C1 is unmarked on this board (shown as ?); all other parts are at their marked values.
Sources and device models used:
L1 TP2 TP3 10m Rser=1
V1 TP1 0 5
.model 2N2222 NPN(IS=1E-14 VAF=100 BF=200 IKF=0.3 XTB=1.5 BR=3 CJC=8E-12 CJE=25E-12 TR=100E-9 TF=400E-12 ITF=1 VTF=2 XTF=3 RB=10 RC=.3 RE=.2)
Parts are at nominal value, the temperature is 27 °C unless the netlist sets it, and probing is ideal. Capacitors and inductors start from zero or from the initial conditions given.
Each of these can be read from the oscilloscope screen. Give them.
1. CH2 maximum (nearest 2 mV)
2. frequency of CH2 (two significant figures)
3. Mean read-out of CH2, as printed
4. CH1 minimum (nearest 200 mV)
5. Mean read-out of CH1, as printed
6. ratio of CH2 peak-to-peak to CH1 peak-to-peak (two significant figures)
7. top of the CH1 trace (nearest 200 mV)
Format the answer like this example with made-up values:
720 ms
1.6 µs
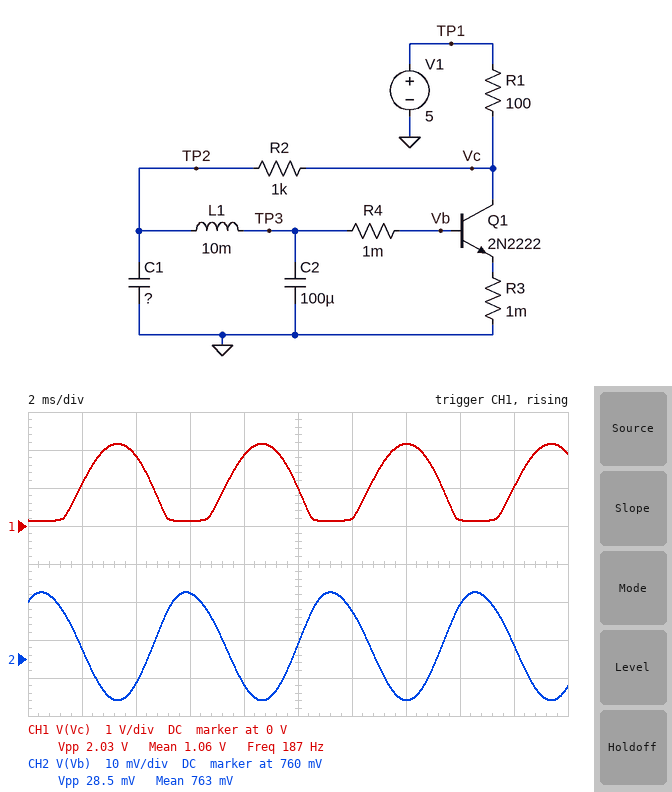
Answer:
778 mV
190 Hz
763 mV
200 mV
1.06 V
0.014
2.2 V
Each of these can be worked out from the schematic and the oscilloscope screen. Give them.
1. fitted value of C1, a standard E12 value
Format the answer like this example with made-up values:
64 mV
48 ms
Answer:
270 µF
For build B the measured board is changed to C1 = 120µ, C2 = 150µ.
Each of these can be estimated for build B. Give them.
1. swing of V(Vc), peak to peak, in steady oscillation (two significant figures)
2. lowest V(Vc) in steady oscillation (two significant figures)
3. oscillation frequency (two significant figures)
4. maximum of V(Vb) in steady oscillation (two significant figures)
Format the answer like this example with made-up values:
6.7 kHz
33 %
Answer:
3.4 V
88 mV
200 Hz
800 mV
